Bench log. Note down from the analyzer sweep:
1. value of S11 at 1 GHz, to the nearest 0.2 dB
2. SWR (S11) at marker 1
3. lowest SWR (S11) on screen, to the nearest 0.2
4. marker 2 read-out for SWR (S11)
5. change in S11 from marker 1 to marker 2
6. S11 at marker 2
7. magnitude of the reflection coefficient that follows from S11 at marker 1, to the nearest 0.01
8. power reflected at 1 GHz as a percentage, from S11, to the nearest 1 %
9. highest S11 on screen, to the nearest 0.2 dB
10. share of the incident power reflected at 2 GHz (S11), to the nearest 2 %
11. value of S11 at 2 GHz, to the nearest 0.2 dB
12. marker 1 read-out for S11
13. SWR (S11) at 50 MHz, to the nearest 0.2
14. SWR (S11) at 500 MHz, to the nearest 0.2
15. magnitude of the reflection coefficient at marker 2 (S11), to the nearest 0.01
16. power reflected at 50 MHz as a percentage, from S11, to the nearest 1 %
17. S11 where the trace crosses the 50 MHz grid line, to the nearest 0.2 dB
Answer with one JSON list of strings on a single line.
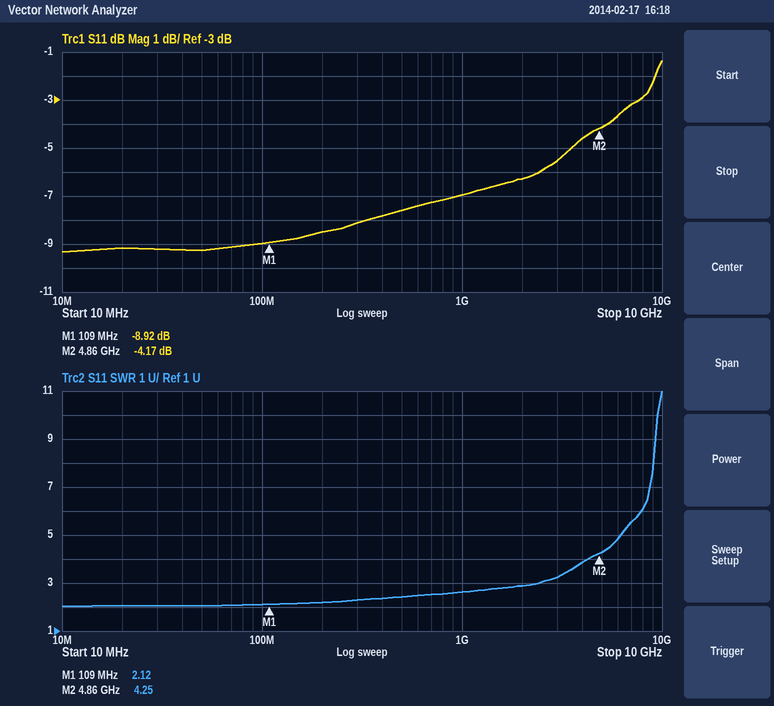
["-7.0 dB", "2.12", "2.0", "4.25", "4.75 dB", "-4.17 dB", "0.36", "20 %", "-1.4 dB", "24 %", "-6.2 dB", "-8.92 dB", "2.0", "2.4", "0.62", "12 %", "-9.2 dB"]
